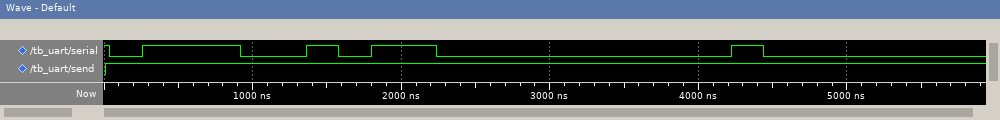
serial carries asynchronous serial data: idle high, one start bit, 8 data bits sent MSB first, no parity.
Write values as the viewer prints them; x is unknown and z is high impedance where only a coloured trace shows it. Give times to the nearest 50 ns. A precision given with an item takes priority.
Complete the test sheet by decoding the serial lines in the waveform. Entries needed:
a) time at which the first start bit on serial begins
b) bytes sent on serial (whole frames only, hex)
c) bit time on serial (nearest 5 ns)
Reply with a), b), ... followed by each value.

a) 0 ns
b) E5, 00
c) 220 ns
